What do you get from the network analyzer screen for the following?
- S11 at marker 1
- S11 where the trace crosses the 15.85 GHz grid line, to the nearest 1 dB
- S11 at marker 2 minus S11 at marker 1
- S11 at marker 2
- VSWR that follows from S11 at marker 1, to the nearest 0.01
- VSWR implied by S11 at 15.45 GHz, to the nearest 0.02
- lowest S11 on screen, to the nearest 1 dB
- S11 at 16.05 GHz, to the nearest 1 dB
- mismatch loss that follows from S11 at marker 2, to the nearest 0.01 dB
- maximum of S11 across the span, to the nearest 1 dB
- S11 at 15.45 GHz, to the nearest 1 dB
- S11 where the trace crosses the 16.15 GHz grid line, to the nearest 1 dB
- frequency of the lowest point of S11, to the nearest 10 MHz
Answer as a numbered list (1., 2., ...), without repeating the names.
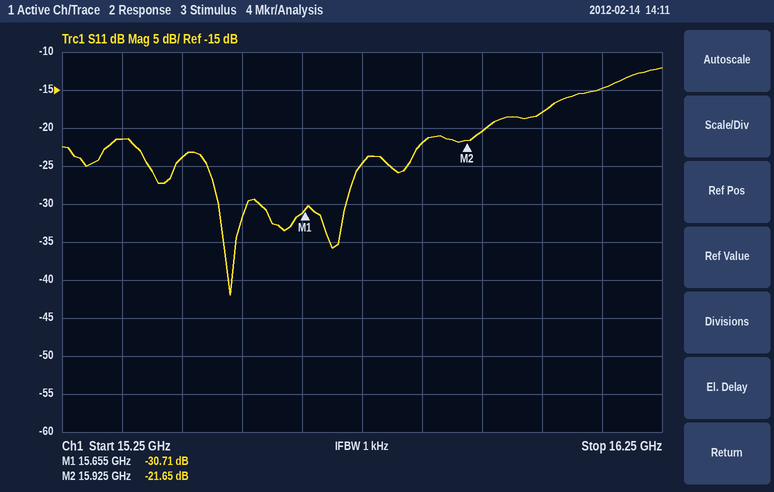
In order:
1. -30.71 dB
2. -22 dB
3. 9.06 dB
4. -21.65 dB
5. 1.06
6. 1.14
7. -42 dB
8. -18 dB
9. 0.03 dB
10. -12 dB
11. -24 dB
12. -15 dB
13. 15.53 GHz
